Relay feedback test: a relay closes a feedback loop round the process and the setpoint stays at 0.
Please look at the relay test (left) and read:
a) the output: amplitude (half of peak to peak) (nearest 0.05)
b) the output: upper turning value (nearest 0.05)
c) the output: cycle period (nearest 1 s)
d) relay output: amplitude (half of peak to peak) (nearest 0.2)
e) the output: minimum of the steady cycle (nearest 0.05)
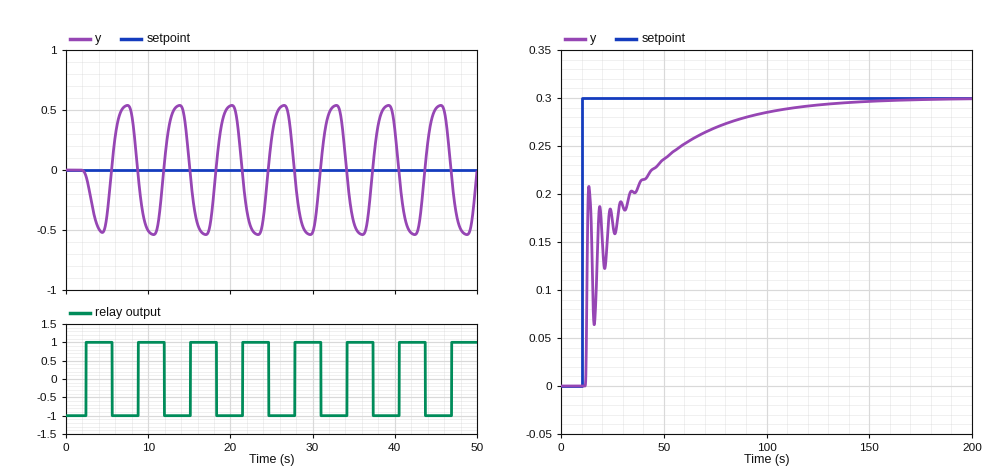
0.55
0.55
6 s
1.0
-0.55
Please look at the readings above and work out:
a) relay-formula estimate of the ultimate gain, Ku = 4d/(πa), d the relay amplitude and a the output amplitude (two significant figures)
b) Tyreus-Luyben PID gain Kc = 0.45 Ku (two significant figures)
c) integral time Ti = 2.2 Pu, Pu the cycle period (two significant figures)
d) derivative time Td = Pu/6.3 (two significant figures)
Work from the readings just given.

2.3
1.0
13 s
0.95 s
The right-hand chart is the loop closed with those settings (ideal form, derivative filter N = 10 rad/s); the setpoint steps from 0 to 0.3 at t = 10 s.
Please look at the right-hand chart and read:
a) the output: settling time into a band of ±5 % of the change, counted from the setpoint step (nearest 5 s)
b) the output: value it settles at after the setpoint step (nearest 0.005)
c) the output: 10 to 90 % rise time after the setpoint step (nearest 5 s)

90 s
0.300
65 s
